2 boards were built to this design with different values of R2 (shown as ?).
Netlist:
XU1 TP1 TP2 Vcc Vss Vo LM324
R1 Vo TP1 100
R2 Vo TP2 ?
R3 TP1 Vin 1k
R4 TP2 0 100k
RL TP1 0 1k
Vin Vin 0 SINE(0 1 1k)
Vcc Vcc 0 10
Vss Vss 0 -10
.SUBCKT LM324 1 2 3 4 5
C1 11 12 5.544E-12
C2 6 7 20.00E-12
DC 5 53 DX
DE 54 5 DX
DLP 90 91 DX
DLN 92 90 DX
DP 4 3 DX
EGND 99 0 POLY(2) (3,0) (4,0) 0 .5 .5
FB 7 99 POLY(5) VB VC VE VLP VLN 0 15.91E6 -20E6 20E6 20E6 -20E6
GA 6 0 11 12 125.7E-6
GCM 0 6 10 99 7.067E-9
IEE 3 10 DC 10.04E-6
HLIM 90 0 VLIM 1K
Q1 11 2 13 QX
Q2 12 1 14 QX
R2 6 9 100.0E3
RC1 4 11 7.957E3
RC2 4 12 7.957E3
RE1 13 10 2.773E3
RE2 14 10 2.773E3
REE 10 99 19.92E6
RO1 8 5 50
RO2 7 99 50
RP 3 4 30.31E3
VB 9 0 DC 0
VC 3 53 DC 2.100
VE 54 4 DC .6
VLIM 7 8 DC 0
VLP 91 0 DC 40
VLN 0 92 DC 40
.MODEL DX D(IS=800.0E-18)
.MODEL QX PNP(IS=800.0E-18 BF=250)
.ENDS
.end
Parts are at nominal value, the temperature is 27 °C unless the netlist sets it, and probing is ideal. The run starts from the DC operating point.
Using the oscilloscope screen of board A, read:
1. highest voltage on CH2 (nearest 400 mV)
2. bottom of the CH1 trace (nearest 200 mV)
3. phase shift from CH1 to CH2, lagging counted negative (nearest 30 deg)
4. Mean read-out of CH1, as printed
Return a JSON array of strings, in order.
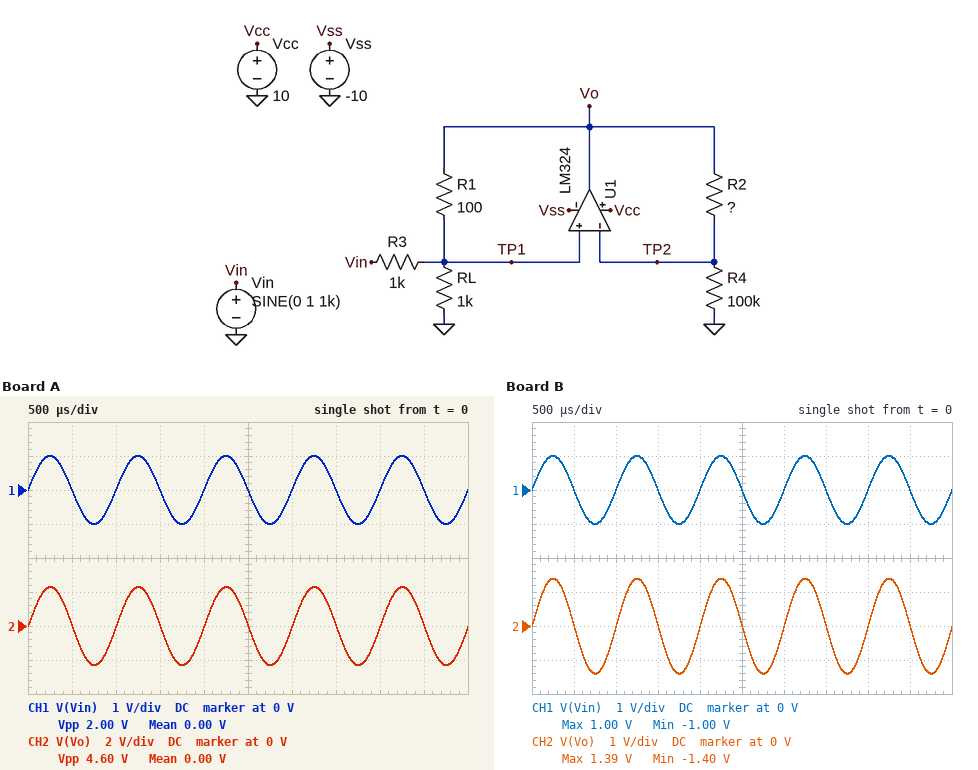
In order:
["2.4 V", "-1.0 V", "0 deg", "0.00 V"]
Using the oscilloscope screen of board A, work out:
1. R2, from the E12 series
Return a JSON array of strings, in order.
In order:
["15 kΩ"]
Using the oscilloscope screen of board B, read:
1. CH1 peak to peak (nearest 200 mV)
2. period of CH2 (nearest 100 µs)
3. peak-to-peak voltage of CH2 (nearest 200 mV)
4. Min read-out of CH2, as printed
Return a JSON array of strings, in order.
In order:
["2.0 V", "1.0 ms", "2.8 V", "-1.40 V"]
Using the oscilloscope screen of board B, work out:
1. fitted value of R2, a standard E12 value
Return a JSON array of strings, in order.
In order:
["12 kΩ"]
